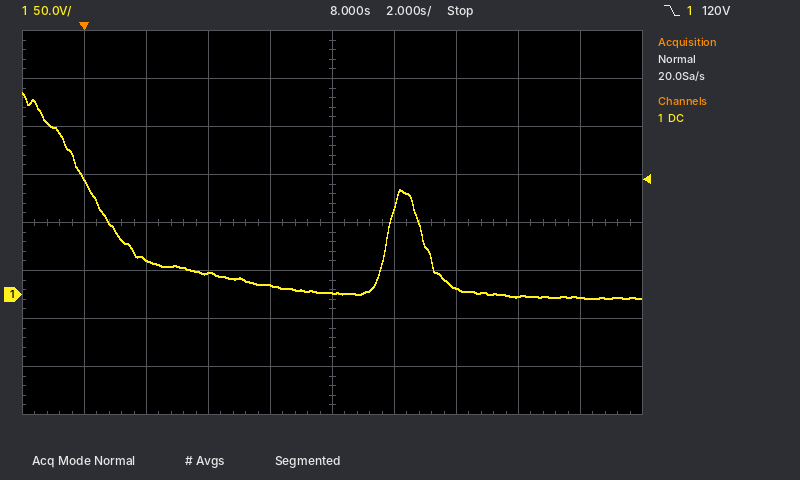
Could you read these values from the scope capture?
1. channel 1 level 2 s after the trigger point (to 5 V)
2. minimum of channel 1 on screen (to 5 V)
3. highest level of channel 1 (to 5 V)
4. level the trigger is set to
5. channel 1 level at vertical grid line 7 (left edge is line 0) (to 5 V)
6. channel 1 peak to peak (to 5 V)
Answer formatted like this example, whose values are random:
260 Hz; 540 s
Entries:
35 V; -5 V; 210 V; 120 V; 5 V; 215 V
